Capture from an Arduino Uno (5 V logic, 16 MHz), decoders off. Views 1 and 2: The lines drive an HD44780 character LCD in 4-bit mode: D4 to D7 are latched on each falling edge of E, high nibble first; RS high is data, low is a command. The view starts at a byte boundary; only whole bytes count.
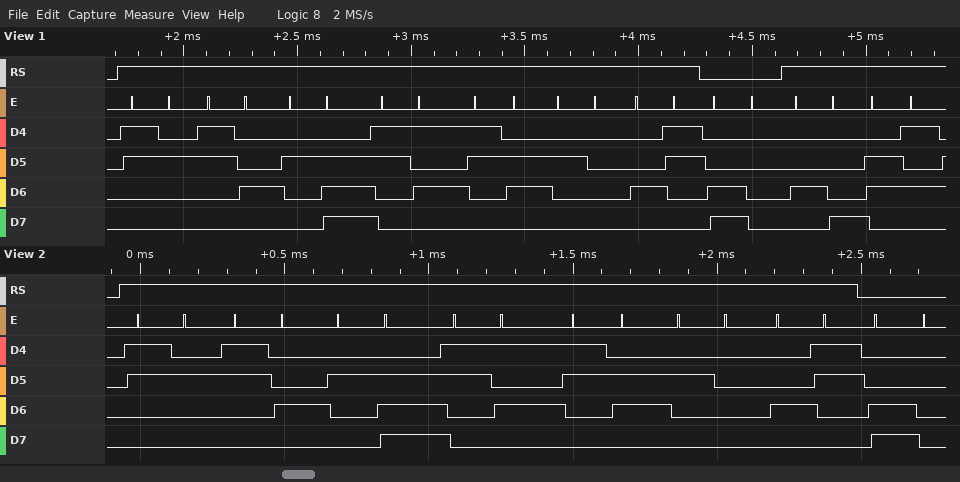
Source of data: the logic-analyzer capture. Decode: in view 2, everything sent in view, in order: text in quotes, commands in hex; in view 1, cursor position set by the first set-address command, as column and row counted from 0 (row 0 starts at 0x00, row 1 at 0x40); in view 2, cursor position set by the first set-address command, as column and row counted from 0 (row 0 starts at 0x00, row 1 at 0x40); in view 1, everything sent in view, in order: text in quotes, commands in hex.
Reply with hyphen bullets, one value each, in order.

- "24.56 C" 0xC0
- column 0, row 1
- column 0, row 1
- "24.56 C" 0xC0 "He"
